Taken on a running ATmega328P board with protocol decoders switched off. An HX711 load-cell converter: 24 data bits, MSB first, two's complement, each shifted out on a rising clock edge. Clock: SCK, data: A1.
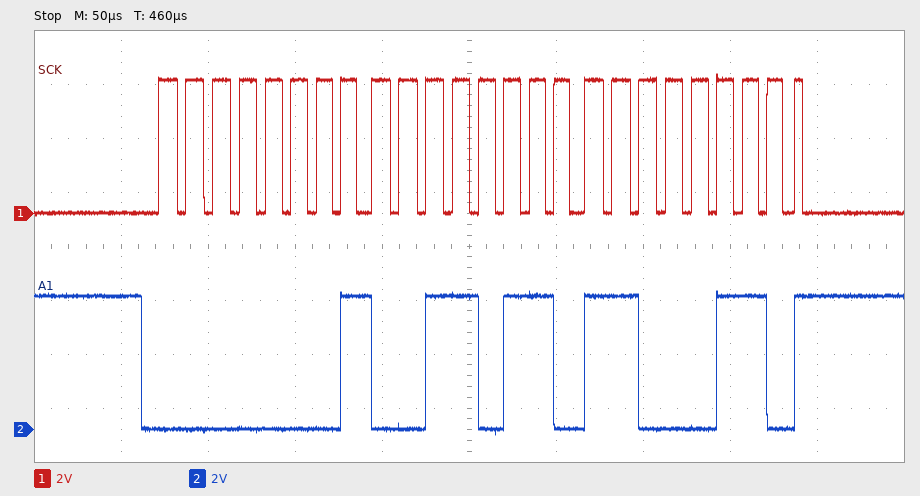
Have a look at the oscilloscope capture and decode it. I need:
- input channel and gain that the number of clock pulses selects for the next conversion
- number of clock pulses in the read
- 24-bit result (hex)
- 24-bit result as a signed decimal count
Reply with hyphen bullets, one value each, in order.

- channel A, gain 128
- 25
- 0x0136C6
- 79558
